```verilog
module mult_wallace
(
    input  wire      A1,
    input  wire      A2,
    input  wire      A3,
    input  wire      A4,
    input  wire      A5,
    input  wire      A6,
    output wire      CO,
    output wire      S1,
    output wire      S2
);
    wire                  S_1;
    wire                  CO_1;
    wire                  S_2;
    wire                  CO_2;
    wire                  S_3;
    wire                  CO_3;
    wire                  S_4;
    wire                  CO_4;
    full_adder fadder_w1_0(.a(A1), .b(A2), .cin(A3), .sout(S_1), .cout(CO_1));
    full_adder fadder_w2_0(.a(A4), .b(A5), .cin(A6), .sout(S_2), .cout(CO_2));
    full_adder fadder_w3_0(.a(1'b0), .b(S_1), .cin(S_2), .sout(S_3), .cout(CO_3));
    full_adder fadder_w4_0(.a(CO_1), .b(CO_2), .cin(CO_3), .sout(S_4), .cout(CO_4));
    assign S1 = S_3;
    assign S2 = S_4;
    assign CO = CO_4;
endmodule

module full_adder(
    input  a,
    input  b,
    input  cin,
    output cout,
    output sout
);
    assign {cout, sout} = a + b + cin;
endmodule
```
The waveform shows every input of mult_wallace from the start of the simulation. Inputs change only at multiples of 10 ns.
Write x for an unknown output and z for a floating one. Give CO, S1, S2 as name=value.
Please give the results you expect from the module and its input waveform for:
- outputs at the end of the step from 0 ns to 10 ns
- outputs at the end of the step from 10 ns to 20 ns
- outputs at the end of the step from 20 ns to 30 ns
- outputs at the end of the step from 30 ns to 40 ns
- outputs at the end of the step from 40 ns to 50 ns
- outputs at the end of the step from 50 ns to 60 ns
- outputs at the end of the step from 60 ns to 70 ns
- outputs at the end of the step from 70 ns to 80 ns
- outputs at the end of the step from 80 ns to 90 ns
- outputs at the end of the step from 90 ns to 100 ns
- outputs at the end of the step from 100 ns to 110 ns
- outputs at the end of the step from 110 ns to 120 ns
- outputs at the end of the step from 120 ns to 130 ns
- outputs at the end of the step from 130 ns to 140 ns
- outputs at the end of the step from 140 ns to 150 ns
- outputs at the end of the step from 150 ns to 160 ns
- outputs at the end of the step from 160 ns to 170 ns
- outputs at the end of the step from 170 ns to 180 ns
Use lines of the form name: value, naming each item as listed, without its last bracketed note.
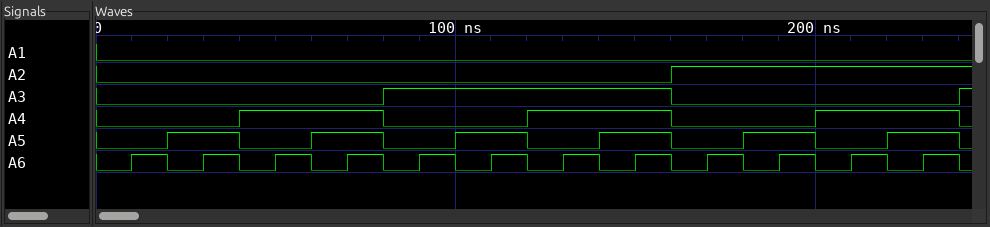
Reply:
outputs at the end of the step from 0 ns to 10 ns: CO=0, S1=0, S2=0
outputs at the end of the step from 10 ns to 20 ns: CO=0, S1=1, S2=0
outputs at the end of the step from 20 ns to 30 ns: CO=0, S1=1, S2=0
outputs at the end of the step from 30 ns to 40 ns: CO=0, S1=0, S2=1
outputs at the end of the step from 40 ns to 50 ns: CO=0, S1=1, S2=0
outputs at the end of the step from 50 ns to 60 ns: CO=0, S1=0, S2=1
outputs at the end of the step from 60 ns to 70 ns: CO=0, S1=0, S2=1
outputs at the end of the step from 70 ns to 80 ns: CO=0, S1=1, S2=1
outputs at the end of the step from 80 ns to 90 ns: CO=0, S1=1, S2=0
outputs at the end of the step from 90 ns to 100 ns: CO=0, S1=0, S2=1
outputs at the end of the step from 100 ns to 110 ns: CO=0, S1=0, S2=1
outputs at the end of the step from 110 ns to 120 ns: CO=0, S1=1, S2=1
outputs at the end of the step from 120 ns to 130 ns: CO=0, S1=0, S2=1
outputs at the end of the step from 130 ns to 140 ns: CO=0, S1=1, S2=1
outputs at the end of the step from 140 ns to 150 ns: CO=0, S1=1, S2=1
outputs at the end of the step from 150 ns to 160 ns: CO=1, S1=0, S2=0
outputs at the end of the step from 160 ns to 170 ns: CO=0, S1=1, S2=0
outputs at the end of the step from 170 ns to 180 ns: CO=0, S1=0, S2=1
